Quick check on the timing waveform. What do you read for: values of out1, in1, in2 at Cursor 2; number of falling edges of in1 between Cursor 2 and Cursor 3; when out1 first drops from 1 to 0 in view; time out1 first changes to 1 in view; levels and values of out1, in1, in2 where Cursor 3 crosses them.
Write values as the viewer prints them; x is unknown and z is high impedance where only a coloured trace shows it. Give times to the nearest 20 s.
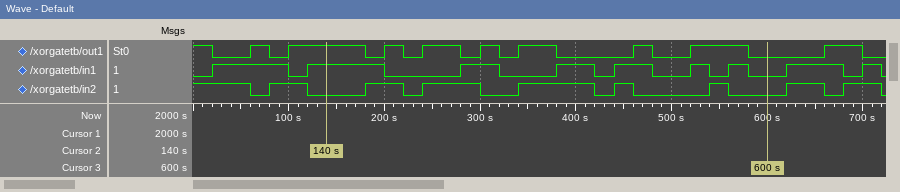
out1=1, in1=1, in2=0
6
20 s
60 s
out1=0, in1=0, in2=0
